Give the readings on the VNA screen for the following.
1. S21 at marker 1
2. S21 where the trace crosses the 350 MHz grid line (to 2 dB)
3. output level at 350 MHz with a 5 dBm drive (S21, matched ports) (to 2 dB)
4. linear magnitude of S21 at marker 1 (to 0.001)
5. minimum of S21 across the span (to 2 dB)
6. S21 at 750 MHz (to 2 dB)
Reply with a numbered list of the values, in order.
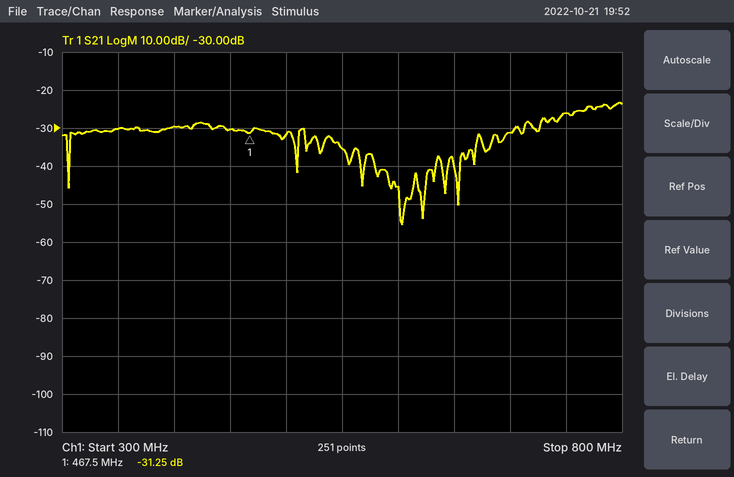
1. -31.25 dB
2. -30 dB
3. -26 dBm
4. 0.027
5. -56 dB
6. -26 dB
